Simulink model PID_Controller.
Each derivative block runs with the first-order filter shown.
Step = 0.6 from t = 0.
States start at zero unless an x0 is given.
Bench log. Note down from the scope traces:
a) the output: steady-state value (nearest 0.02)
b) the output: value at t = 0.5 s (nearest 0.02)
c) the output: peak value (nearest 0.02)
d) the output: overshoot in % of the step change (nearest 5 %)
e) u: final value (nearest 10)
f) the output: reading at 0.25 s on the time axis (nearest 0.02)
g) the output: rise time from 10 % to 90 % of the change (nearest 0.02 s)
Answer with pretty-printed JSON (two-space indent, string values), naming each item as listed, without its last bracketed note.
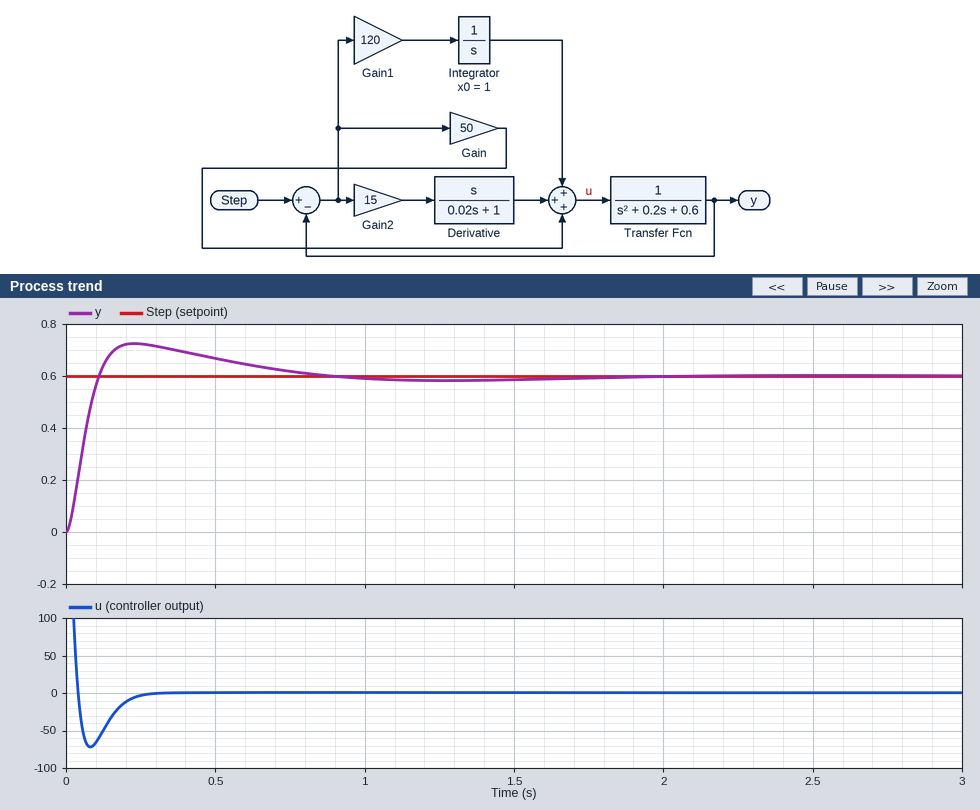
{
  "the output: steady-state value": "0.60",
  "the output: value at t = 0.5 s": "0.66",
  "the output: peak value": "0.72",
  "the output: overshoot in % of the step change": "20 %",
  "u: final value": "0",
  "the output: reading at 0.25 s on the time axis": "0.72",
  "the output: rise time from 10 % to 90 % of the change": "0.08 s"
}
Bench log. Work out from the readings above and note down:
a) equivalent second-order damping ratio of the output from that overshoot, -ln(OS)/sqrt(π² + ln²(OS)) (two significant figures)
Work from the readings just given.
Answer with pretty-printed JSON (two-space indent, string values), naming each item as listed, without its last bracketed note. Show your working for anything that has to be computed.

{
  "equivalent second-order damping ratio of the output from that overshoot, -ln(OS)/sqrt(π² + ln²(OS))": "ln(0.2) = -1.609; 1.609 / sqrt(9.870 + 2.590) = 0.46"
}
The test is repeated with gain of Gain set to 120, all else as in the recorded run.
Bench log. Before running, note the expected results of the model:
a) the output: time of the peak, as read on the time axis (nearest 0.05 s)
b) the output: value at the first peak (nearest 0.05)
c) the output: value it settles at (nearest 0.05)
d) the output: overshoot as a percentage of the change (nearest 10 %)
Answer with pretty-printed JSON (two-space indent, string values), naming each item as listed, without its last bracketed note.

{
  "the output: time of the peak, as read on the time axis": "0.15 s",
  "the output: value at the first peak": "0.80",
  "the output: value it settles at": "0.60",
  "the output: overshoot as a percentage of the change": "30 %"
}
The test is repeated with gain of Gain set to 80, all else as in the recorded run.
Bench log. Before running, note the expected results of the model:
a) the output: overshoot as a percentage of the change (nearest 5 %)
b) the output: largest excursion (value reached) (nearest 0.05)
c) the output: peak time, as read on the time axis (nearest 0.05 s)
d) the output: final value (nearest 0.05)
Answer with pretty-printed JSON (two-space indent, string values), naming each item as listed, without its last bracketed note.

{
  "the output: overshoot as a percentage of the change": "25 %",
  "the output: largest excursion (value reached)": "0.75",
  "the output: peak time, as read on the time axis": "0.20 s",
  "the output: final value": "0.60"
}
